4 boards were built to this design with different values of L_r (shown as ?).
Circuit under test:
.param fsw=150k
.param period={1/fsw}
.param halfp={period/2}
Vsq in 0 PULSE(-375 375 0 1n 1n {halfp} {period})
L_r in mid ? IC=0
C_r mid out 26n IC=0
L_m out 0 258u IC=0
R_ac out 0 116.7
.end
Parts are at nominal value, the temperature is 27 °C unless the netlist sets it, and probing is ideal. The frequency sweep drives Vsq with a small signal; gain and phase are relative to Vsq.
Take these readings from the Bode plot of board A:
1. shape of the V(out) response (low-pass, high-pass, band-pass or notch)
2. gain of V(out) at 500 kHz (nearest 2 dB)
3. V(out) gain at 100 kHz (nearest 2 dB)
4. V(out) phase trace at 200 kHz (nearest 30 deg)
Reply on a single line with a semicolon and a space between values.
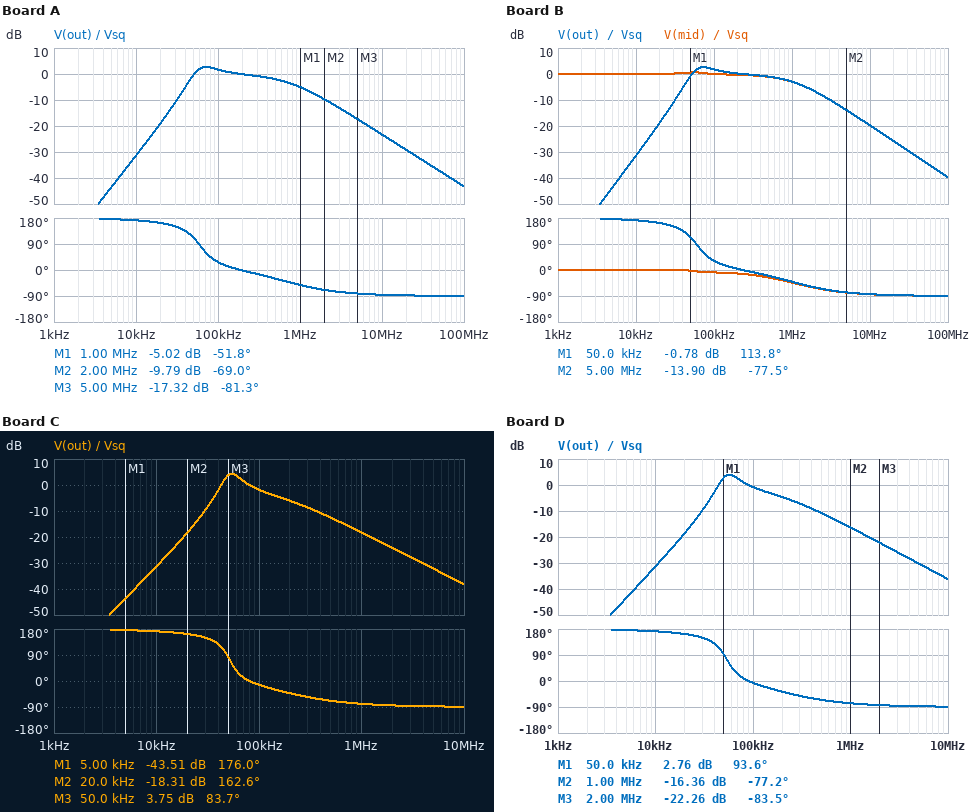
band-pass; -2 dB; 2 dB; 0 deg
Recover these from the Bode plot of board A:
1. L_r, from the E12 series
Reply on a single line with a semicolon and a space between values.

27 µH
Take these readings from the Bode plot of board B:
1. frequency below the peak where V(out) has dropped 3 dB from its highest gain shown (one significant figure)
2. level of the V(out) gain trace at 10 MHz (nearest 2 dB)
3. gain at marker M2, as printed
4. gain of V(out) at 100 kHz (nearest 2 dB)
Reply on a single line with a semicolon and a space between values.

50 kHz; -20 dB; -13.90 dB; 2 dB
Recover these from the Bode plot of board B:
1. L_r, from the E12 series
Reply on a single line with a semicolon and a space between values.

18 µH
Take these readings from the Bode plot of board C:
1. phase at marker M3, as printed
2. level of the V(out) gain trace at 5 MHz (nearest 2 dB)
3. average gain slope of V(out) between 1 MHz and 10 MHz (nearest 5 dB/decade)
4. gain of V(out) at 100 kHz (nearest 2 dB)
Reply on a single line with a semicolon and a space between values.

83.7 deg; -32 dB; -20 dB/decade; -2 dB
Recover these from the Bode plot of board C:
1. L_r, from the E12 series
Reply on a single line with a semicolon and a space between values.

150 µH
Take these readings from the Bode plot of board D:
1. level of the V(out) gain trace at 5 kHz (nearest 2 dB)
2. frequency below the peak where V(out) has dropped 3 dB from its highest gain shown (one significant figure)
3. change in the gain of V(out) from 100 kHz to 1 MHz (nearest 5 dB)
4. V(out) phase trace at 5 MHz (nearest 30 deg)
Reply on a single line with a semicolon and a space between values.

-44 dB; 50 kHz; -15 dB; -90 deg
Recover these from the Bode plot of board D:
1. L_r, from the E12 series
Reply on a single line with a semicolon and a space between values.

120 µH
